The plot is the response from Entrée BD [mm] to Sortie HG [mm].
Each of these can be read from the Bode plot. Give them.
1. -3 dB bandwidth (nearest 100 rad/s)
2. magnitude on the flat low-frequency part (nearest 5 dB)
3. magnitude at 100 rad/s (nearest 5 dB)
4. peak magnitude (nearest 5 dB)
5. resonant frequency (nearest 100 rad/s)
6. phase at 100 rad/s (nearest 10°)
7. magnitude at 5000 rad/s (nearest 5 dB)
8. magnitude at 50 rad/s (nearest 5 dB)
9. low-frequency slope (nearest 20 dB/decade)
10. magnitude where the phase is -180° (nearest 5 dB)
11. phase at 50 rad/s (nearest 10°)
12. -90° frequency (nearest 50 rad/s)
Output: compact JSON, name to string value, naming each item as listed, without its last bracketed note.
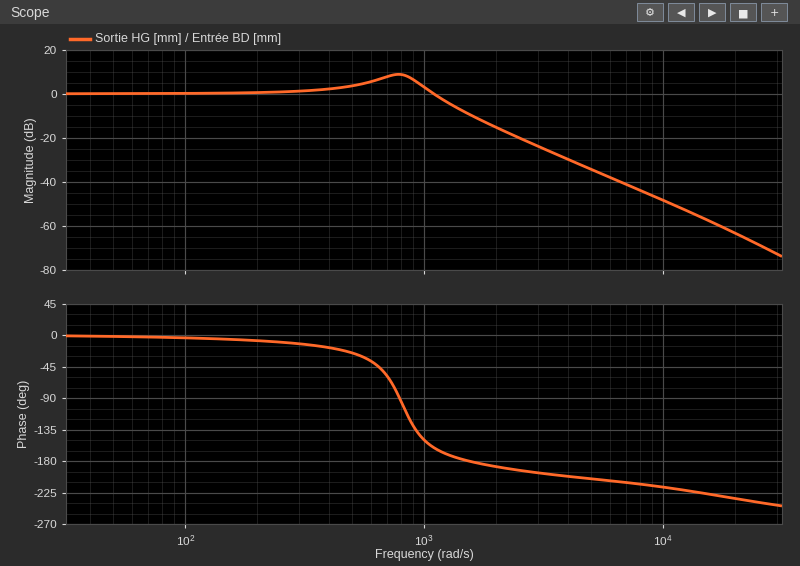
{"-3 dB bandwidth": "1200 rad/s", "magnitude on the flat low-frequency part": "0 dB", "magnitude at 100 rad/s": "0 dB", "peak magnitude": "10 dB", "resonant frequency": "800 rad/s", "phase at 100 rad/s": "0°", "magnitude at 5000 rad/s": "-35 dB", "magnitude at 50 rad/s": "0 dB", "low-frequency slope": "0 dB/decade", "magnitude where the phase is -180°": "-10 dB", "phase at 50 rad/s": "0°", "-90° frequency": "800 rad/s"}
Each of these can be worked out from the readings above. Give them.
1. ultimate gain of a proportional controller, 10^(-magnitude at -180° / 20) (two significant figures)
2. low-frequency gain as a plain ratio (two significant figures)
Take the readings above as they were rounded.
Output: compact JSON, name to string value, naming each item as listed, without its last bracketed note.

{"ultimate gain of a proportional controller, 10^(-magnitude at -180° / 20)": "3.2", "low-frequency gain as a plain ratio": "1.0"}
